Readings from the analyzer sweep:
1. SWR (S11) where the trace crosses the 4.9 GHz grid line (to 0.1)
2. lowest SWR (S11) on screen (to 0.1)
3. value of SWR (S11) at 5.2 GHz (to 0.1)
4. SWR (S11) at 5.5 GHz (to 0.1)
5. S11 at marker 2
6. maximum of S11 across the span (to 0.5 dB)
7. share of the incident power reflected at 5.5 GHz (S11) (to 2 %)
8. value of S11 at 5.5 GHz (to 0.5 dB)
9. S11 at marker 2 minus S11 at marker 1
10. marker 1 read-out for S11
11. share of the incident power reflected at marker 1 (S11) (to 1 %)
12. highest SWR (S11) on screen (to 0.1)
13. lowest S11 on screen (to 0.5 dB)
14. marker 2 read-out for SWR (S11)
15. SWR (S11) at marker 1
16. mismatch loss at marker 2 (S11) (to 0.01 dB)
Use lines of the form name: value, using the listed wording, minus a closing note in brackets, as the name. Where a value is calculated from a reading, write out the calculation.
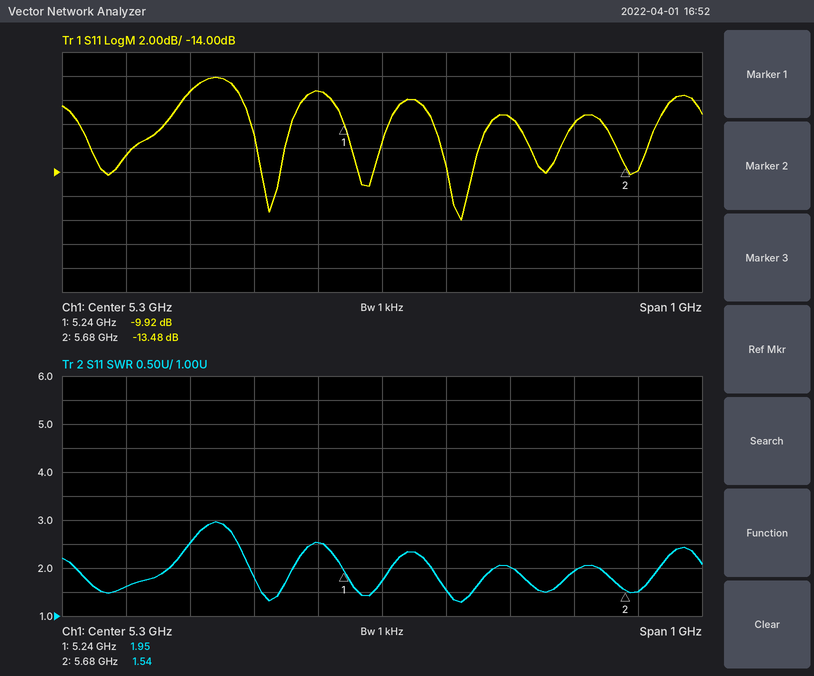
SWR (S11) where the trace crosses the 4.9 GHz grid line: 1.6
lowest SWR (S11) on screen: 1.3
value of SWR (S11) at 5.2 GHz: 2.5
SWR (S11) at 5.5 GHz: 2.0
S11 at marker 2: -13.48 dB
maximum of S11 across the span: -6.0 dB
share of the incident power reflected at 5.5 GHz (S11): 10^(-9.5/10) ≈ 11.2 %, so 12 % to the nearest 2 %
value of S11 at 5.5 GHz: -9.5 dB
S11 at marker 2 minus S11 at marker 1: -13.48 − (-9.92) = -3.56 dB
marker 1 read-out for S11: -9.92 dB
share of the incident power reflected at marker 1 (S11): 10^(-9.92/10) ≈ 10 %
highest SWR (S11) on screen: 3.0
lowest S11 on screen: -18.0 dB
marker 2 read-out for SWR: 1.54
SWR (S11) at marker 1: 1.95
mismatch loss at marker 2 (S11): −10 log10(1 − 10^(-13.48/10)) ≈ 0.20 dB
